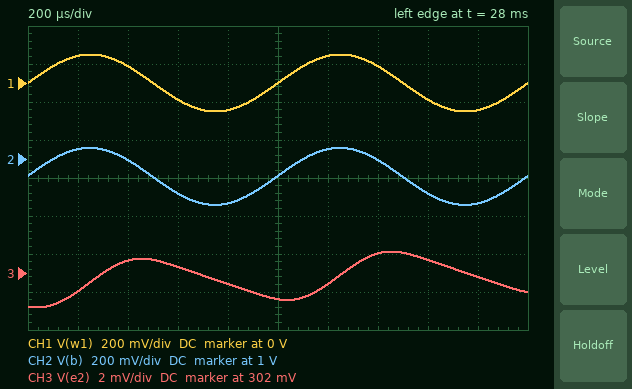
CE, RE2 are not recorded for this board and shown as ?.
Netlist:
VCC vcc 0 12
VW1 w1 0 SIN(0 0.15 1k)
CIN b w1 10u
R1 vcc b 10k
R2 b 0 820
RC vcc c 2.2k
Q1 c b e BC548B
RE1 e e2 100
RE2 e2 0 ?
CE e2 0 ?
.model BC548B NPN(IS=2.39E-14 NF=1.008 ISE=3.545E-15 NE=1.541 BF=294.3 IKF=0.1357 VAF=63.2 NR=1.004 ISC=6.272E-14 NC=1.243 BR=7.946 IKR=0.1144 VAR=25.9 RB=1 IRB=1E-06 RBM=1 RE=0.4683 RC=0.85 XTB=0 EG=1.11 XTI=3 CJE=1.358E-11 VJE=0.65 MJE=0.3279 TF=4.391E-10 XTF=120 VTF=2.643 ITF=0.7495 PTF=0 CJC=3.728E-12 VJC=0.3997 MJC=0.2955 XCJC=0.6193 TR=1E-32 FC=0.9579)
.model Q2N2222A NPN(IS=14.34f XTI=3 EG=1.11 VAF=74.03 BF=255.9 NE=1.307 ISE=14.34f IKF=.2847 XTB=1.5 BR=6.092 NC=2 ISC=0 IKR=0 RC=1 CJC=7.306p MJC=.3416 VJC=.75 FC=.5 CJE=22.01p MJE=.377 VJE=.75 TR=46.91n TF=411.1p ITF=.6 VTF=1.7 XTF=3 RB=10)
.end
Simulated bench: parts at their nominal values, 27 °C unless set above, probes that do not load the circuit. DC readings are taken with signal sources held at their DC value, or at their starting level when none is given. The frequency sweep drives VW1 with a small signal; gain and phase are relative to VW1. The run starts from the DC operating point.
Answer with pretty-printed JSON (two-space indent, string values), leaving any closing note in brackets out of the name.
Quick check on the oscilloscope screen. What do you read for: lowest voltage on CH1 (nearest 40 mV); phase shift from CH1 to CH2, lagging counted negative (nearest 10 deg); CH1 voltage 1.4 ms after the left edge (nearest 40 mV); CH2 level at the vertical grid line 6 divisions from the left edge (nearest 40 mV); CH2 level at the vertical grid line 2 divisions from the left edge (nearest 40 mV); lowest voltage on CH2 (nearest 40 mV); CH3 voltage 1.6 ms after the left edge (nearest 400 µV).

{
  "lowest voltage on CH1": "-160 mV",
  "phase shift from CH1 to CH2, lagging counted negative": "0 deg",
  "CH1 voltage 1.4 ms after the left edge": "80 mV",
  "CH2 level at the vertical grid line 6 divisions from the left edge": "1.04 V",
  "CH2 level at the vertical grid line 2 divisions from the left edge": "1.00 V",
  "lowest voltage on CH2": "760 mV",
  "CH3 voltage 1.6 ms after the left edge": "302.8 mV"
}
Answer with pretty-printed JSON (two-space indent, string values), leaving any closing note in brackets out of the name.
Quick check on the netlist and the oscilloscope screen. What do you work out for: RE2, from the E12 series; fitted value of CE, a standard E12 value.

{
  "RE2, from the E12 series": "820 Ω",
  "fitted value of CE, a standard E12 value": "82 µF"
}
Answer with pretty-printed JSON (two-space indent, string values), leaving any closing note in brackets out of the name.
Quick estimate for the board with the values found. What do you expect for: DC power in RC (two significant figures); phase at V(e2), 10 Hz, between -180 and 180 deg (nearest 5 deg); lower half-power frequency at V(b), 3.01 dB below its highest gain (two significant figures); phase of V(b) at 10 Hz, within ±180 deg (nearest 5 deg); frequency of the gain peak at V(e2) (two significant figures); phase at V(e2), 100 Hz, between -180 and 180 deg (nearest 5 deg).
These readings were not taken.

{
  "DC power in RC": "240 µW",
  "phase at V(e2), 10 Hz, between -180 and 180 deg": "25 deg",
  "lower half-power frequency at V(b), 3.01 dB below its highest gain": "21 Hz",
  "phase of V(b) at 10 Hz, within ±180 deg": "65 deg",
  "frequency of the gain peak at V(e2)": "17 Hz",
  "phase at V(e2), 100 Hz, between -180 and 180 deg": "-70 deg"
}
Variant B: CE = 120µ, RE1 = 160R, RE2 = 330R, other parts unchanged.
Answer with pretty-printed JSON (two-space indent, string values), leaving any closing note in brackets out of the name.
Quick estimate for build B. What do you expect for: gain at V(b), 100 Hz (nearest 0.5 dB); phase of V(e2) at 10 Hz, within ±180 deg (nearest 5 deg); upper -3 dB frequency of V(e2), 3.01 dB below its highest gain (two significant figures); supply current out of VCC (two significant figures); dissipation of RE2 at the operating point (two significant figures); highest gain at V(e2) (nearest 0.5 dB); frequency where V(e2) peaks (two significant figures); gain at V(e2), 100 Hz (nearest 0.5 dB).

{
  "gain at V(b), 100 Hz": "0 dB",
  "phase of V(e2) at 10 Hz, within ±180 deg": "20 deg",
  "upper -3 dB frequency of V(e2), 3.01 dB below its highest gain": "38 Hz",
  "supply current out of VCC": "1.7 mA",
  "dissipation of RE2 at the operating point": "110 µW",
  "highest gain at V(e2)": "-14.0 dB",
  "frequency where V(e2) peaks": "15 Hz",
  "gain at V(e2), 100 Hz": "-24.0 dB"
}
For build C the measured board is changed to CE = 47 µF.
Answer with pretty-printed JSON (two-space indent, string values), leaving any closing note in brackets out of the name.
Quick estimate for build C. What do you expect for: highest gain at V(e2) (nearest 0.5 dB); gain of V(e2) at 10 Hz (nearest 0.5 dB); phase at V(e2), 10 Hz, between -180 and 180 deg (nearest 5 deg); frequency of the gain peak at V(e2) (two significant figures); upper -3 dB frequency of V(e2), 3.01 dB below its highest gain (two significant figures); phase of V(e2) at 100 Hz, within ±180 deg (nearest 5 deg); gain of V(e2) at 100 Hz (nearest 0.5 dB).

{
  "highest gain at V(e2)": "-7.5 dB",
  "gain of V(e2) at 10 Hz": "-10.0 dB",
  "phase at V(e2), 10 Hz, between -180 and 180 deg": "40 deg",
  "frequency of the gain peak at V(e2)": "22 Hz",
  "upper -3 dB frequency of V(e2), 3.01 dB below its highest gain": "53 Hz",
  "phase of V(e2) at 100 Hz, within ±180 deg": "-65 deg",
  "gain of V(e2) at 100 Hz": "-15.0 dB"
}
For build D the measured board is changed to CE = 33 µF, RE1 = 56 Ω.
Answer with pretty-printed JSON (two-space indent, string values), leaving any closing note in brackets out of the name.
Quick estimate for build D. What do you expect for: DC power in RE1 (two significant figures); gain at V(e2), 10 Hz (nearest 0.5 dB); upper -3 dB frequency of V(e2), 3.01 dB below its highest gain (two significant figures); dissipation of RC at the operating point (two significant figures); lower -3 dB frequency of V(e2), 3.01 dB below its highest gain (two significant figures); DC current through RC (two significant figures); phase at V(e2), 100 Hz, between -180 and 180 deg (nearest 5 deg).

{
  "DC power in RE1": "6.7 µW",
  "gain at V(e2), 10 Hz": "-9.0 dB",
  "upper -3 dB frequency of V(e2), 3.01 dB below its highest gain": "75 Hz",
  "dissipation of RC at the operating point": "260 µW",
  "lower -3 dB frequency of V(e2), 3.01 dB below its highest gain": "12 Hz",
  "DC current through RC": "340 µA",
  "phase at V(e2), 100 Hz, between -180 and 180 deg": "-55 deg"
}
